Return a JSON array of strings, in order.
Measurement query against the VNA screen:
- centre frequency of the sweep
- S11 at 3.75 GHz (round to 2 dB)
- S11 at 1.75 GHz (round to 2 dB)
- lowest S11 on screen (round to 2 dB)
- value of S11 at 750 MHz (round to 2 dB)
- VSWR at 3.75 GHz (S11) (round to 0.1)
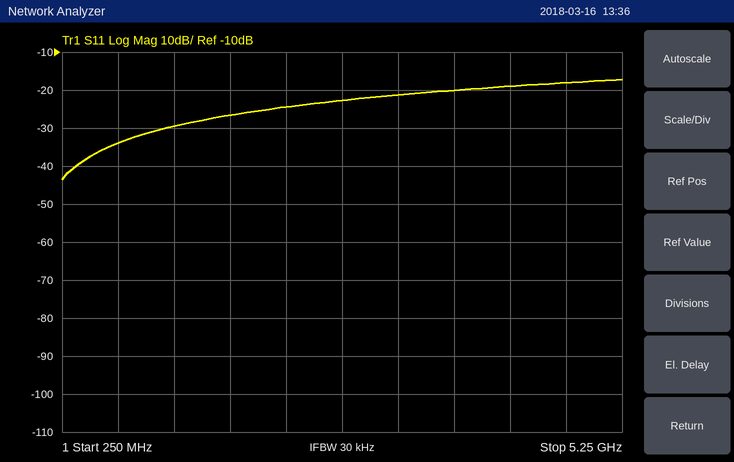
["2.75 GHz", "-20 dB", "-26 dB", "-44 dB", "-34 dB", "1.2"]
